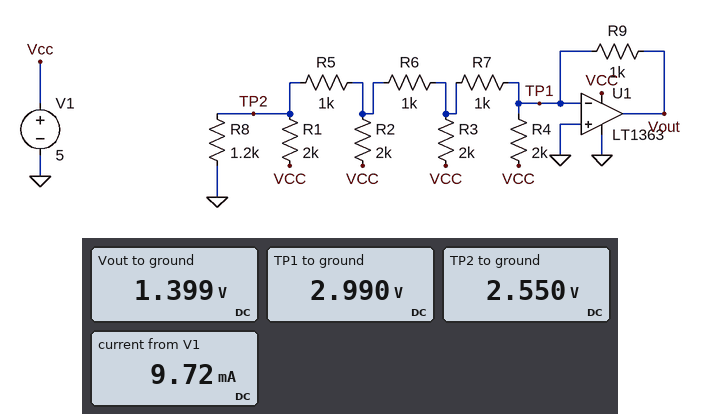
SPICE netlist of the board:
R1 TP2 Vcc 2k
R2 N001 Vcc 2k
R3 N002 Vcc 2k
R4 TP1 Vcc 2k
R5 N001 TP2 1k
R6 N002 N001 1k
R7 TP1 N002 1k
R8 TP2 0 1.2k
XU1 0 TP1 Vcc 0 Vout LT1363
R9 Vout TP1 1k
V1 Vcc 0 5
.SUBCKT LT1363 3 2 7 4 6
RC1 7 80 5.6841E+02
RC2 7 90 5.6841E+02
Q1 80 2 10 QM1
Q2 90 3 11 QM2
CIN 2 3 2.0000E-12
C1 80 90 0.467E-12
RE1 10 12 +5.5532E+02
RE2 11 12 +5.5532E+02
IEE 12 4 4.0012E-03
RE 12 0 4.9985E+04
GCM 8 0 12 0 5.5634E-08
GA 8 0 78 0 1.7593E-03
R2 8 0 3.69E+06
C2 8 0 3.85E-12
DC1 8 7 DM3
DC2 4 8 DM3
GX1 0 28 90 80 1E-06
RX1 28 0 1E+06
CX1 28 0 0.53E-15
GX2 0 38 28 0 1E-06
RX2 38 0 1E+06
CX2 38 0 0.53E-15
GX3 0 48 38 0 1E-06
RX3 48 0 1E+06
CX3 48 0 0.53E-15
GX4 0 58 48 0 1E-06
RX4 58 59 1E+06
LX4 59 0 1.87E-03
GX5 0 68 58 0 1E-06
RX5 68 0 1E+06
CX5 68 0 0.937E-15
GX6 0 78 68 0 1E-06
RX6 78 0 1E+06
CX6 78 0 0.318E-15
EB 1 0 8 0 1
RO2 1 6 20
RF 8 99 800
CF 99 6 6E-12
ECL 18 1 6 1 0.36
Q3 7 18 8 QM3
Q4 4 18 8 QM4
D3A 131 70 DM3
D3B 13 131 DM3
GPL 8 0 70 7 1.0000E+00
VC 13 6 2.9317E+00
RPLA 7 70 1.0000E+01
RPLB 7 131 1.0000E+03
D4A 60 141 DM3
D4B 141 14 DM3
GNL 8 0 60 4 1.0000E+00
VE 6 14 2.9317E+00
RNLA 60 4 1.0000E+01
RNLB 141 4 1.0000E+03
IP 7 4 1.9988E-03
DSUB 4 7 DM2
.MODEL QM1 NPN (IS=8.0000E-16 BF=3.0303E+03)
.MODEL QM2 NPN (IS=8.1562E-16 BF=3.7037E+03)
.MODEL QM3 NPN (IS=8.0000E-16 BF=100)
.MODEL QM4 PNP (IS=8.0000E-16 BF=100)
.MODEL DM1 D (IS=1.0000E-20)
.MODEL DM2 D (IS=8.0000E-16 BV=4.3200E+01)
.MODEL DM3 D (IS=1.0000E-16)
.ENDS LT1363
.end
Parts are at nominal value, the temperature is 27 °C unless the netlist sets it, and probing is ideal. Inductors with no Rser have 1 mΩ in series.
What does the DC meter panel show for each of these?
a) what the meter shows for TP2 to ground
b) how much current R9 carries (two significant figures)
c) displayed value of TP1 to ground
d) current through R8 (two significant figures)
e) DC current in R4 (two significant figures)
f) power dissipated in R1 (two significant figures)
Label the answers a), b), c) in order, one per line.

a) 2.550 V
b) 1.6 mA
c) 2.990 V
d) 2.1 mA
e) 1.0 mA
f) 3.0 mW
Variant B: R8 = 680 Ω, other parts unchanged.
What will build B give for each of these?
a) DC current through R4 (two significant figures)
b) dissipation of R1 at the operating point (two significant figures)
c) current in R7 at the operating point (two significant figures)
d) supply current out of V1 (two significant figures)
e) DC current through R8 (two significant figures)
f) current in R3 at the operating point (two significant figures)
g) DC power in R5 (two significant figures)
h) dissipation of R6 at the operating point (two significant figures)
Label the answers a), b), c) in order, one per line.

a) 1.0 mA
b) 4.8 mW
c) 490 µA
d) 10 mA
e) 2.8 mA
f) 790 µA
g) 1.5 mW
h) 87 µW
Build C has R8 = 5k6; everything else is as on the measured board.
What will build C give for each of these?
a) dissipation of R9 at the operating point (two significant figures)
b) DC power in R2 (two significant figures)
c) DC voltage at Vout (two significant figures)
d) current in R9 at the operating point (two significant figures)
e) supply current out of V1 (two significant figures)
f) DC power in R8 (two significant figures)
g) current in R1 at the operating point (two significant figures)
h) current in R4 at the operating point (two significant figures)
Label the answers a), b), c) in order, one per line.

a) 3.0 mW
b) 360 µW
c) 1.4 V
d) 1.7 mA
e) 8.4 mA
f) 2.8 mW
g) 520 µA
h) 940 µA
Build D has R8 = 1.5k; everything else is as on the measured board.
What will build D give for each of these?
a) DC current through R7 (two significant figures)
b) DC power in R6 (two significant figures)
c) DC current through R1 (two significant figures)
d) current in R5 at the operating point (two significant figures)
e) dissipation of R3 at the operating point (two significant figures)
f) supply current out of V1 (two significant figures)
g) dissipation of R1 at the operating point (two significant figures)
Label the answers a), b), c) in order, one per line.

a) 620 µA
b) 3.6 µW
c) 1.1 mA
d) 770 µA
e) 930 µW
f) 9.5 mA
g) 2.4 mW
